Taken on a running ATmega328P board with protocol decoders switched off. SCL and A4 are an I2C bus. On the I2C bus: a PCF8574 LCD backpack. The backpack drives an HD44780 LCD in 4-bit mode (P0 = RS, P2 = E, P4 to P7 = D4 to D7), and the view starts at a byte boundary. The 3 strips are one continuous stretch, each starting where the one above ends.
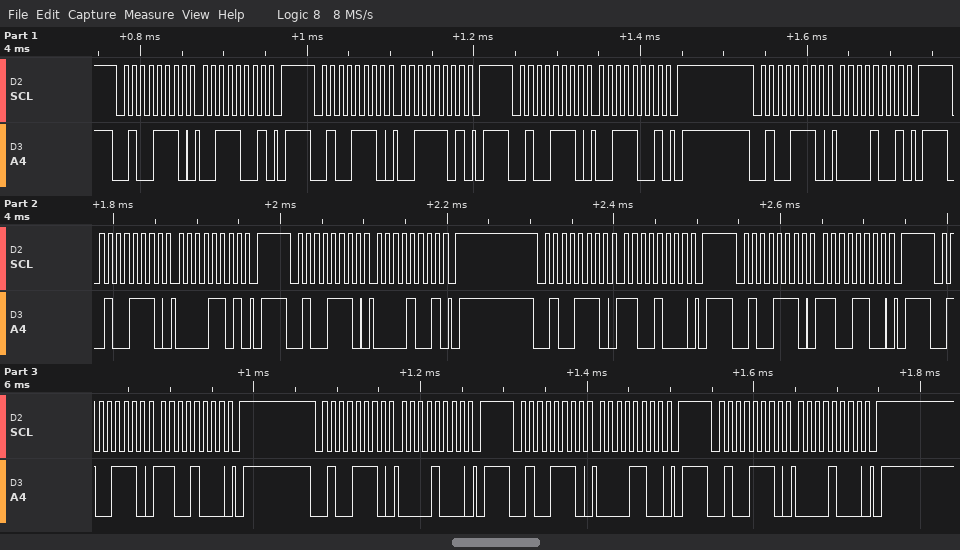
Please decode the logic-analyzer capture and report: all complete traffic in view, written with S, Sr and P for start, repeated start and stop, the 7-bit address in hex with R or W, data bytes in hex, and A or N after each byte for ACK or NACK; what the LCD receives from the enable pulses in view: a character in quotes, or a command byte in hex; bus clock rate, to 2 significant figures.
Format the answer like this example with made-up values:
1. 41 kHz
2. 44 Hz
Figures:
1. S 27W A 39 A P S 27W A 3D A P S 27W A 39 A P S 27W A 09 A P S 27W A 0D A P S 27W A 09 A P S 27W A C8 A P S 27W A CC A P S 27W A C8 A P S 27W A 08 A P S 27W A 0C A P S 27W A 08 A P
2. '0' 0xC0
3. 100 kHz
